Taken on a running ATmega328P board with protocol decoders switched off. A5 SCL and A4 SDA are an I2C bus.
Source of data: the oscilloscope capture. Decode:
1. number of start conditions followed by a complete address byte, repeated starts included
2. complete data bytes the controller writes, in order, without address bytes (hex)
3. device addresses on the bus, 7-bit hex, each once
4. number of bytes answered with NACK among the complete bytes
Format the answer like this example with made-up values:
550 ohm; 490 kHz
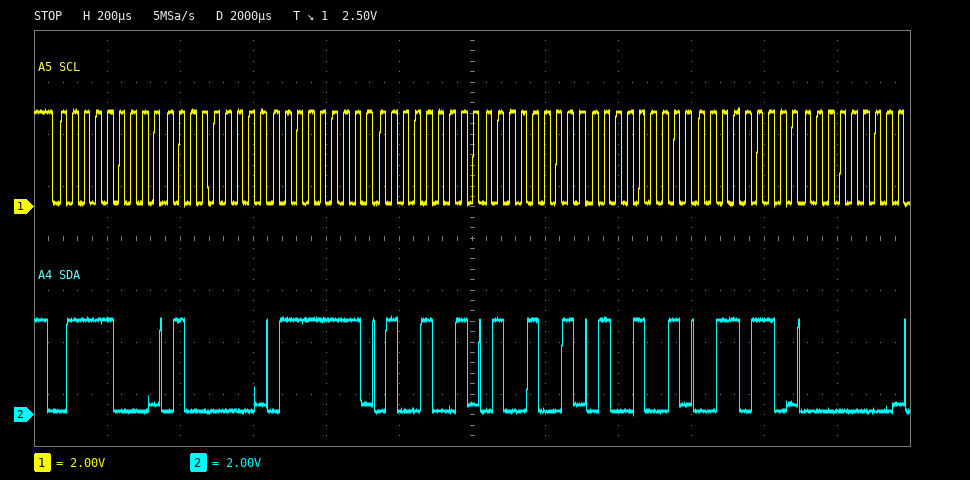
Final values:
1; 40 7F 49 49 49 36 00; 0x3C; 0
